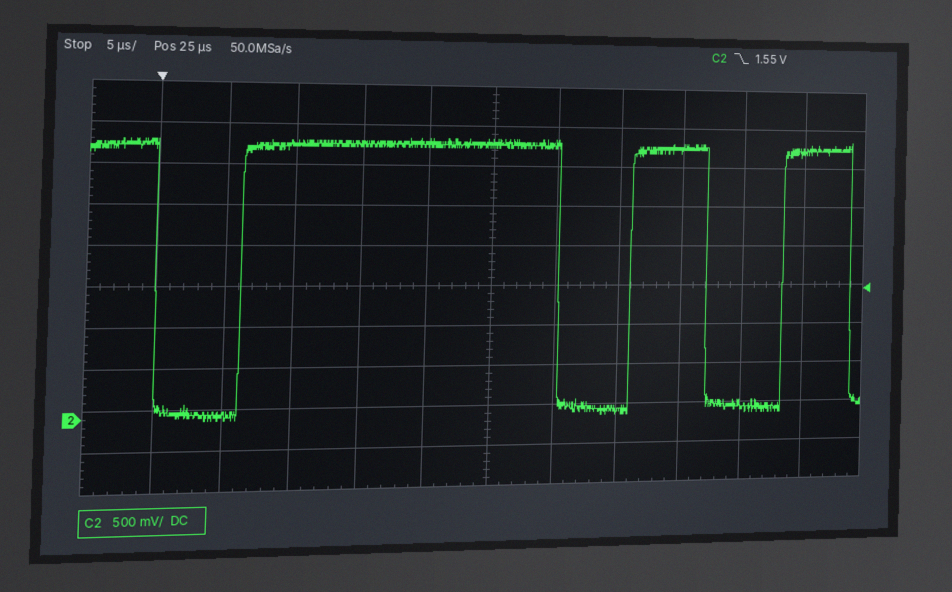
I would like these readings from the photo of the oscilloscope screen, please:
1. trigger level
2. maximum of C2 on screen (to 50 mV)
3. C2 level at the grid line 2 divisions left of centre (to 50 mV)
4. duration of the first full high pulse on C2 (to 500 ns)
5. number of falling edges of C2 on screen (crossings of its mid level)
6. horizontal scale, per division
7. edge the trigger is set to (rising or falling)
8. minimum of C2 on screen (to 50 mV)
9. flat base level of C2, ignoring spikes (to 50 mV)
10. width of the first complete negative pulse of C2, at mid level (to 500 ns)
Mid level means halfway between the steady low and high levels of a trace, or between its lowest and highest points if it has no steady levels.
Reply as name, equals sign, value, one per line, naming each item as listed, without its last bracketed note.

trigger level = 1.55 V
maximum of C2 on screen = 3.45 V
C2 level at the grid line 2 divisions left of centre = 3.35 V
duration of the first full high pulse on C2 = 24.0 µs
number of falling edges of C2 on screen = 4
horizontal scale, per division = 5 µs
edge the trigger is set to = falling
minimum of C2 on screen = -50 mV
flat base level of C2, ignoring spikes = 50 mV
width of the first complete negative pulse of C2, at mid level = 6.0 µs
